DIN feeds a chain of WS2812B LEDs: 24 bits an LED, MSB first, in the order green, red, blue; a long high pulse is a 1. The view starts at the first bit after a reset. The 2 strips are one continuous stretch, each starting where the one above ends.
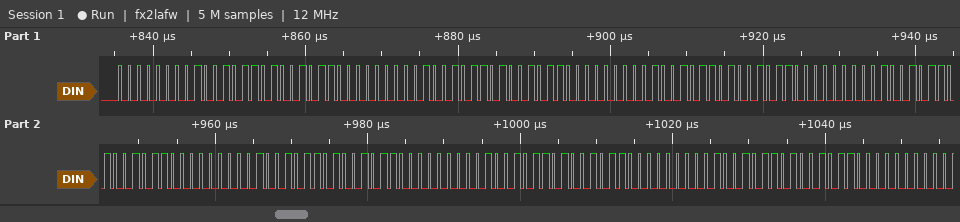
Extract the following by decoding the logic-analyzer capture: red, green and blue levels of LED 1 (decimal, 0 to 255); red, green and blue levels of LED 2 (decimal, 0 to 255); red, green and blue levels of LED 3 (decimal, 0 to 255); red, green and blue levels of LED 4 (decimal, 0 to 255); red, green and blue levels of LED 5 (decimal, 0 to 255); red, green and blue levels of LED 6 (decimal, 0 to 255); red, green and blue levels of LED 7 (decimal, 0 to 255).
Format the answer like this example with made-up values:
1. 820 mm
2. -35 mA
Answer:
1. 150, 0, 150
2. 150, 0, 150
3. 150, 0, 150
4. 150, 0, 150
5. 150, 0, 150
6. 150, 0, 150
7. 150, 0, 150
